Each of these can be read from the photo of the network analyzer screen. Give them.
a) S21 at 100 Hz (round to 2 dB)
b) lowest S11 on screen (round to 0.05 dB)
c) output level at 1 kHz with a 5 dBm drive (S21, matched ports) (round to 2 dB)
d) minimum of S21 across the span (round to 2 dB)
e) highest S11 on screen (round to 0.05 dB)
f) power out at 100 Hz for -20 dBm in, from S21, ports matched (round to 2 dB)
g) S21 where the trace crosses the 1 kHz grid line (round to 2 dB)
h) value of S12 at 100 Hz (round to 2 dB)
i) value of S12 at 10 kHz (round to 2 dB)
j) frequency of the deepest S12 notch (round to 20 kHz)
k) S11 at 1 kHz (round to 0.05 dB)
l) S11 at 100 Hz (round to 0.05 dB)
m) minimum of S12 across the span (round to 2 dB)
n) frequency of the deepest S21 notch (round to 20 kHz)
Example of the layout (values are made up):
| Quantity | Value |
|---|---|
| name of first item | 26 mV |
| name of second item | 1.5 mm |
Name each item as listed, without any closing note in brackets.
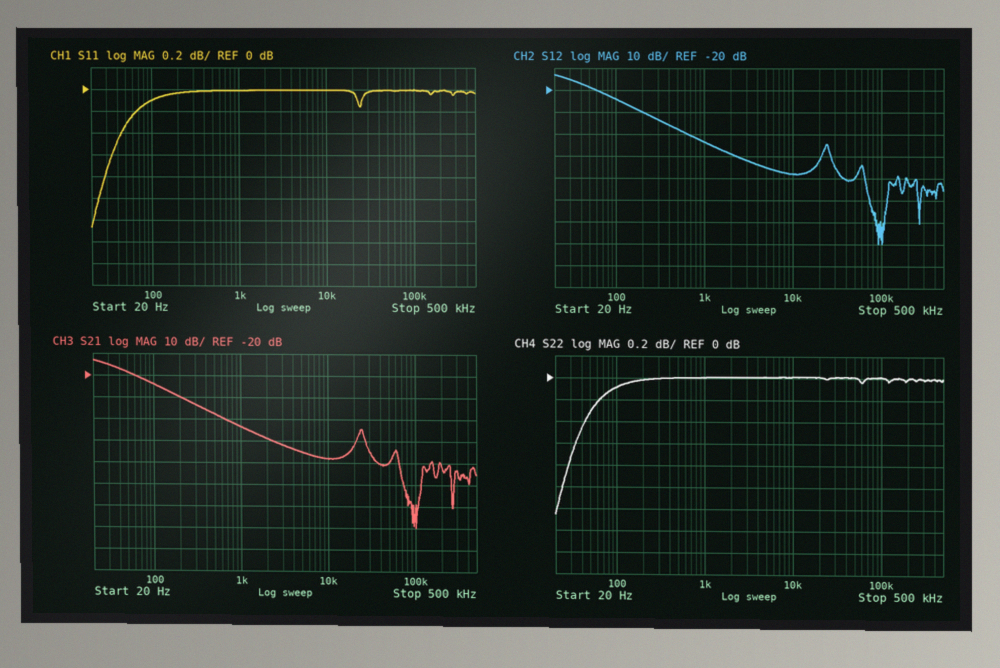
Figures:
| Quantity | Value |
|---|---|
| S21 at 100 Hz | -24 dB |
| lowest S11 on screen | -1.25 dB |
| output level at 1 kHz with a 5 dBm drive (S21, matched ports) | -38 dBm |
| minimum of S21 across the span | -90 dB |
| highest S11 on screen | 0.00 dB |
| power out at 100 Hz for -20 dBm in, from S21, ports matched | -44 dBm |
| S21 where the trace crosses the 1 kHz grid line | -44 dB |
| value of S12 at 100 Hz | -24 dB |
| value of S12 at 10 kHz | -58 dB |
| frequency of the deepest S12 notch | 100 kHz |
| S11 at 1 kHz | 0.00 dB |
| S11 at 100 Hz | -0.10 dB |
| minimum of S12 across the span | -90 dB |
| frequency of the deepest S21 notch | 100 kHz |
